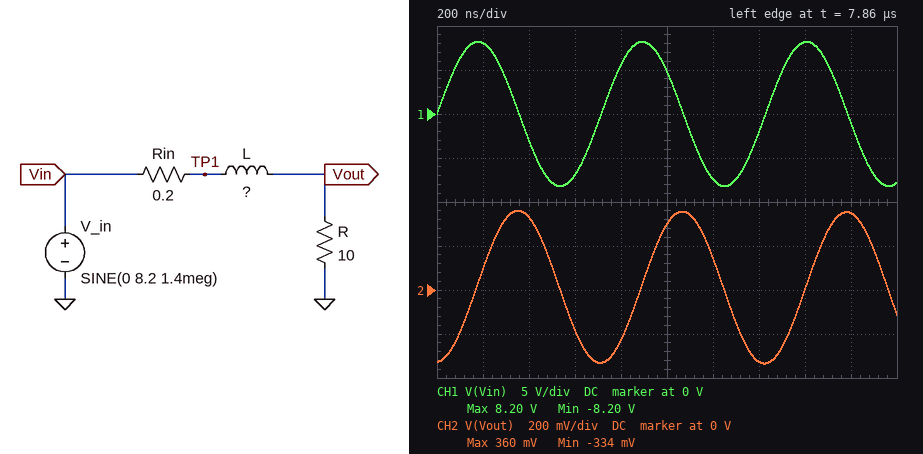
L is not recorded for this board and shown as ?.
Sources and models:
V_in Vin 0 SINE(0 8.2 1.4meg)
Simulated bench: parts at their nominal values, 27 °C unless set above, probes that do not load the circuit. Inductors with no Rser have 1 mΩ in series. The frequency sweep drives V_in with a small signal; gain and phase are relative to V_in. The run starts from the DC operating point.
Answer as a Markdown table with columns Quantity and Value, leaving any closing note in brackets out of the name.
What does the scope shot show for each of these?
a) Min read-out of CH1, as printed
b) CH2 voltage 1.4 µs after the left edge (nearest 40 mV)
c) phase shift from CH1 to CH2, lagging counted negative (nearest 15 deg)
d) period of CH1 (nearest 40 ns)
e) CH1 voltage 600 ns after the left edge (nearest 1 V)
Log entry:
| Quantity | Value |
|---|---|
| Min read-out of CH1, as printed | -8.20 V |
| CH2 voltage 1.4 µs after the left edge | -320 mV |
| phase shift from CH1 to CH2, lagging counted negative | -90 deg |
| period of CH1 | 720 ns |
| CH1 voltage 600 ns after the left edge | -7 V |
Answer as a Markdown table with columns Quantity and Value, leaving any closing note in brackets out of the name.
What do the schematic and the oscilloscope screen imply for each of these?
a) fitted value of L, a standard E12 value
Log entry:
| Quantity | Value |
|---|---|
| fitted value of L, a standard E12 value | 27 µH |
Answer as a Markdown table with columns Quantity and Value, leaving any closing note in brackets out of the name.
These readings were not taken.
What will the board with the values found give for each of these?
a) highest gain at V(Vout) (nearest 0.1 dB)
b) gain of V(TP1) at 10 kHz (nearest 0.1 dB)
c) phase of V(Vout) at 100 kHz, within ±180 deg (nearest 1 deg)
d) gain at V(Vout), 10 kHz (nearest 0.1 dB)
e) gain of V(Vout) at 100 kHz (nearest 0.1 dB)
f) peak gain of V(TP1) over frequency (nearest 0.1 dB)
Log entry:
| Quantity | Value |
|---|---|
| highest gain at V(Vout) | -0.2 dB |
| gain of V(TP1) at 10 kHz | -0.2 dB |
| phase of V(Vout) at 100 kHz, within ±180 deg | -59 deg |
| gain at V(Vout), 10 kHz | -0.3 dB |
| gain of V(Vout) at 100 kHz | -5.9 dB |
| peak gain of V(TP1) over frequency | 0 dB |
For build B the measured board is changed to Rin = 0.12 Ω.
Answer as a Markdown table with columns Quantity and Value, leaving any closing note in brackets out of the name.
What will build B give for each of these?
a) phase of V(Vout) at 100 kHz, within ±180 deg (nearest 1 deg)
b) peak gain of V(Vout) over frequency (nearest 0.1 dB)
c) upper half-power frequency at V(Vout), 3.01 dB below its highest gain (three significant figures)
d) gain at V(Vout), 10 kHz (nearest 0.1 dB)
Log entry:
| Quantity | Value |
|---|---|
| phase of V(Vout) at 100 kHz, within ±180 deg | -59 deg |
| peak gain of V(Vout) over frequency | -0.1 dB |
| upper half-power frequency at V(Vout), 3.01 dB below its highest gain | 59.7 kHz |
| gain at V(Vout), 10 kHz | -0.2 dB |
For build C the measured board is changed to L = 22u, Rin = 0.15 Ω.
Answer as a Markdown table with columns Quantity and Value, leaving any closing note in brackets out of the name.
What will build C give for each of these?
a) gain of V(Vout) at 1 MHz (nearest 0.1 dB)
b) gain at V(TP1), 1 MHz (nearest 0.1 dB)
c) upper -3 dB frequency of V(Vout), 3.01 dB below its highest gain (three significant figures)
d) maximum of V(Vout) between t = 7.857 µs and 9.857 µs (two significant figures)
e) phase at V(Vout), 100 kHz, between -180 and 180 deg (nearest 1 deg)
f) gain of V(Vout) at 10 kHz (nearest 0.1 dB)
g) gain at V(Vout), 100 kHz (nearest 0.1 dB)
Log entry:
| Quantity | Value |
|---|---|
| gain of V(Vout) at 1 MHz | -22.8 dB |
| gain at V(TP1), 1 MHz | 0 dB |
| upper -3 dB frequency of V(Vout), 3.01 dB below its highest gain | 73.4 kHz |
| maximum of V(Vout) between t = 7.857 µs and 9.857 µs | 430 mV |
| phase at V(Vout), 100 kHz, between -180 and 180 deg | -54 deg |
| gain of V(Vout) at 10 kHz | -0.2 dB |
| gain at V(Vout), 100 kHz | -4.7 dB |
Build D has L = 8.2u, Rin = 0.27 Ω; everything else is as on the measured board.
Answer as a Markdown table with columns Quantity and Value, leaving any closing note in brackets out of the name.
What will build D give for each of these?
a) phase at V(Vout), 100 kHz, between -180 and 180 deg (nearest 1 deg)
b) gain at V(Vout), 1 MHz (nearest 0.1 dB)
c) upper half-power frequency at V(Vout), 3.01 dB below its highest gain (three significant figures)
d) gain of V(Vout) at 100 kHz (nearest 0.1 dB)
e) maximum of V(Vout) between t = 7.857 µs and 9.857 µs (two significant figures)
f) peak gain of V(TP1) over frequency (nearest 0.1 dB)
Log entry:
| Quantity | Value |
|---|---|
| phase at V(Vout), 100 kHz, between -180 and 180 deg | -27 deg |
| gain at V(Vout), 1 MHz | -14.4 dB |
| upper half-power frequency at V(Vout), 3.01 dB below its highest gain | 199 kHz |
| gain of V(Vout) at 100 kHz | -1.2 dB |
| maximum of V(Vout) between t = 7.857 µs and 9.857 µs | 1.1 V |
| peak gain of V(TP1) over frequency | 0 dB |
